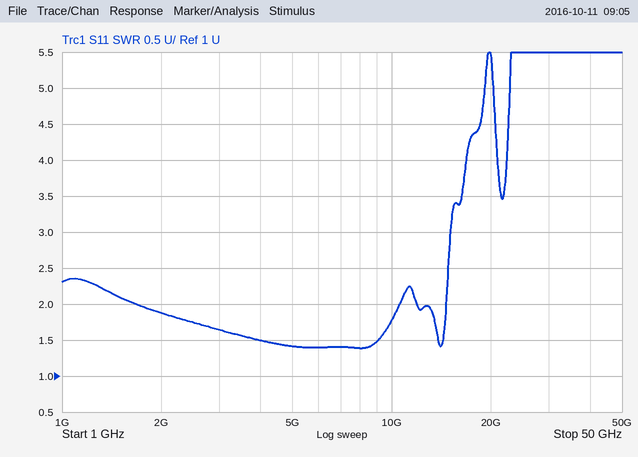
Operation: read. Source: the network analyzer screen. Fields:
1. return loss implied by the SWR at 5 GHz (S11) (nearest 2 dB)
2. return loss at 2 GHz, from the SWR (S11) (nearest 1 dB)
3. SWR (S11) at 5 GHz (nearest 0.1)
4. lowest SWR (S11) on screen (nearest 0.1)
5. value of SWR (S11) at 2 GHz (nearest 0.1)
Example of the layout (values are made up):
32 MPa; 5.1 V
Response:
16 dB; 10 dB; 1.4; 1.4; 1.9
